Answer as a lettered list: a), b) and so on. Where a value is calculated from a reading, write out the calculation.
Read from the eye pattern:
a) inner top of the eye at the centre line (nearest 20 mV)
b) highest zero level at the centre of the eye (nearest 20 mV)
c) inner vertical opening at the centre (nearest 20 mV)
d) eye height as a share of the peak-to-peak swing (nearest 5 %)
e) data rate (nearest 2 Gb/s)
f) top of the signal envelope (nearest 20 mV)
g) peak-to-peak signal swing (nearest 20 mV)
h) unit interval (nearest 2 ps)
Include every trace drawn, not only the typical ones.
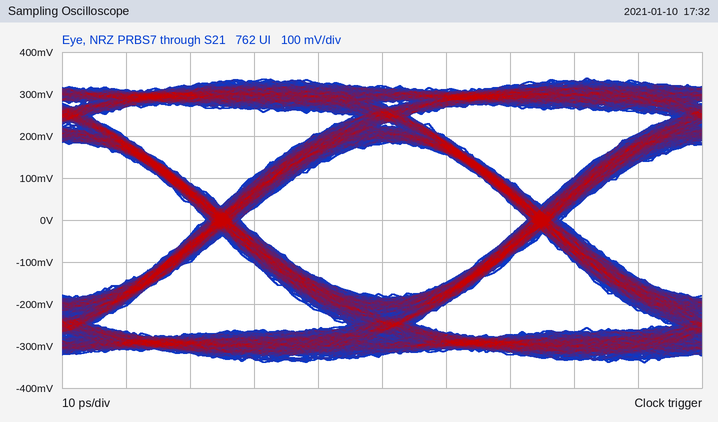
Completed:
a) 180 mV
b) -180 mV
c) 360 mV
d) 360 mV / 680 mV ≈ 52.9 %, so 55 % to the nearest 5 %
e) 20 Gb/s
f) 340 mV
g) 680 mV
h) 50 ps
